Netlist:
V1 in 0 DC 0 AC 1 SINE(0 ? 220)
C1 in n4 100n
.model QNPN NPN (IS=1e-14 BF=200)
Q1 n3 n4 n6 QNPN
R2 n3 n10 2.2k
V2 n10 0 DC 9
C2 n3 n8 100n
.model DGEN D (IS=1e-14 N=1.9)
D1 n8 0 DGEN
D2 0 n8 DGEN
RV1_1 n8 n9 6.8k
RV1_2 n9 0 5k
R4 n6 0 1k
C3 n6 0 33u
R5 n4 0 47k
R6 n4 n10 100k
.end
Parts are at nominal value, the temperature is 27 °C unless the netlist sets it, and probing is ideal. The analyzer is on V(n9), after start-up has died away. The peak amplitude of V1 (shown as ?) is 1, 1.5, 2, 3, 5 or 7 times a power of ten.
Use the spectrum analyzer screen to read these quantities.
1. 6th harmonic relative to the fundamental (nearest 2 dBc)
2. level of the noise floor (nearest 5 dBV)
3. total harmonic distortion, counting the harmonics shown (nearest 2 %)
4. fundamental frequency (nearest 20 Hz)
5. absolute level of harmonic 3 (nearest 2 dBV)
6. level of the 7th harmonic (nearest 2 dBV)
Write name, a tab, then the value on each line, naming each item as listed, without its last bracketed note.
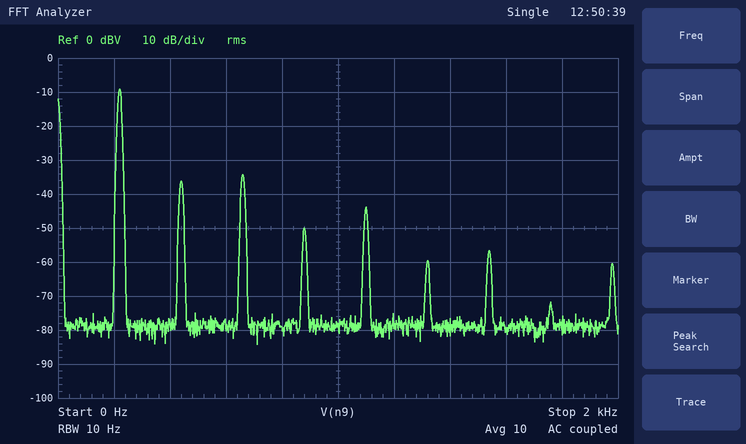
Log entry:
6th harmonic relative to the fundamental	-50 dBc
level of the noise floor	-80 dBV
total harmonic distortion, counting the harmonics shown	8 %
fundamental frequency	220 Hz
absolute level of harmonic 3	-34 dBV
level of the 7th harmonic	-56 dBV
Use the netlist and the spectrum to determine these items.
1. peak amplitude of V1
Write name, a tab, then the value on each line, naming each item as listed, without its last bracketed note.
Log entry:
peak amplitude of V1	50 mV
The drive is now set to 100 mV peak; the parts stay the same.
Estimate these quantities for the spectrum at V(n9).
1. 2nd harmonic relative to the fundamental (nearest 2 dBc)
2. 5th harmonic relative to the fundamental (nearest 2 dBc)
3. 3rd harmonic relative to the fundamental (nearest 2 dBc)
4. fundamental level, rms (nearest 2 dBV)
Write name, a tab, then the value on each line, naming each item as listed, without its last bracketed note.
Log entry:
2nd harmonic relative to the fundamental	-20 dBc
5th harmonic relative to the fundamental	-24 dBc
3rd harmonic relative to the fundamental	-16 dBc
fundamental level, rms	-8 dBV
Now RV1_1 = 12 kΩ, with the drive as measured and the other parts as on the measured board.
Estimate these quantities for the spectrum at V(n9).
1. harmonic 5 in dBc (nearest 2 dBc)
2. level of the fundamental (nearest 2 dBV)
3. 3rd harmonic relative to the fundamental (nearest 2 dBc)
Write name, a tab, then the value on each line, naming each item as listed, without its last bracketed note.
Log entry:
harmonic 5 in dBc	-34 dBc
level of the fundamental	-12 dBV
3rd harmonic relative to the fundamental	-22 dBc
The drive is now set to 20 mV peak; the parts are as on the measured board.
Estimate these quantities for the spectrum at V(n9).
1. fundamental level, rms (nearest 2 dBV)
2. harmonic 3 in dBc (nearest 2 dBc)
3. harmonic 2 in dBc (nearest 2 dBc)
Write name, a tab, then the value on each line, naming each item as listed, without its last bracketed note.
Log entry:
fundamental level, rms	-16 dBV
harmonic 3 in dBc	-58 dBc
harmonic 2 in dBc	-34 dBc
